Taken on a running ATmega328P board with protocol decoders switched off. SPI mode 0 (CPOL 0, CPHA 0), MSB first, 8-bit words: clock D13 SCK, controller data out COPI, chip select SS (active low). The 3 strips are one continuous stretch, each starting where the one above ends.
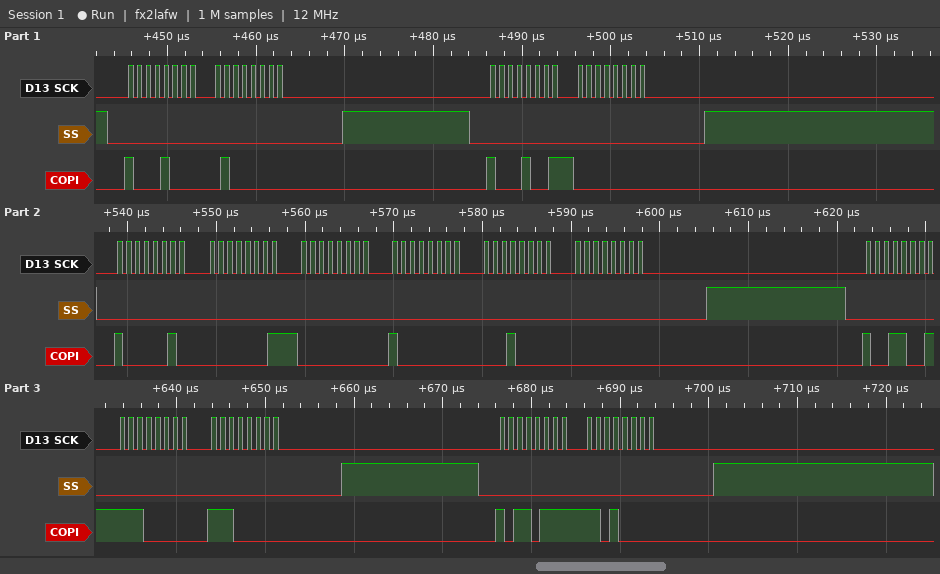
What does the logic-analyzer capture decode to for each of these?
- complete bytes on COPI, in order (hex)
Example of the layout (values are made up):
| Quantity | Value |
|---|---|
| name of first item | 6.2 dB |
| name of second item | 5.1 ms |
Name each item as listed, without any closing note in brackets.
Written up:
| Quantity | Value |
|---|---|
| complete bytes on COPI, in order | 88 40 89 00 82 01 00 80 10 00 99 E0 E0 B7 D0 |
